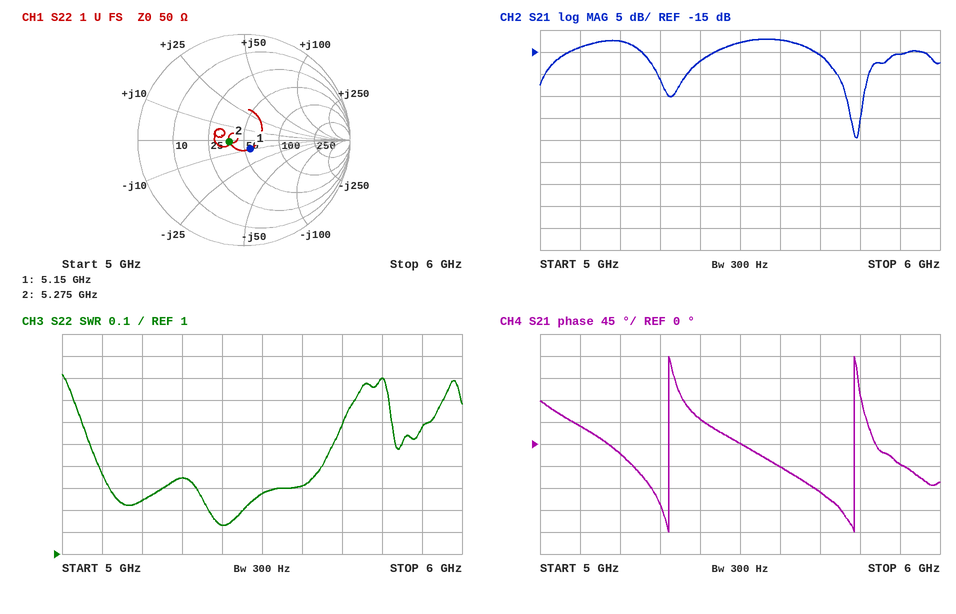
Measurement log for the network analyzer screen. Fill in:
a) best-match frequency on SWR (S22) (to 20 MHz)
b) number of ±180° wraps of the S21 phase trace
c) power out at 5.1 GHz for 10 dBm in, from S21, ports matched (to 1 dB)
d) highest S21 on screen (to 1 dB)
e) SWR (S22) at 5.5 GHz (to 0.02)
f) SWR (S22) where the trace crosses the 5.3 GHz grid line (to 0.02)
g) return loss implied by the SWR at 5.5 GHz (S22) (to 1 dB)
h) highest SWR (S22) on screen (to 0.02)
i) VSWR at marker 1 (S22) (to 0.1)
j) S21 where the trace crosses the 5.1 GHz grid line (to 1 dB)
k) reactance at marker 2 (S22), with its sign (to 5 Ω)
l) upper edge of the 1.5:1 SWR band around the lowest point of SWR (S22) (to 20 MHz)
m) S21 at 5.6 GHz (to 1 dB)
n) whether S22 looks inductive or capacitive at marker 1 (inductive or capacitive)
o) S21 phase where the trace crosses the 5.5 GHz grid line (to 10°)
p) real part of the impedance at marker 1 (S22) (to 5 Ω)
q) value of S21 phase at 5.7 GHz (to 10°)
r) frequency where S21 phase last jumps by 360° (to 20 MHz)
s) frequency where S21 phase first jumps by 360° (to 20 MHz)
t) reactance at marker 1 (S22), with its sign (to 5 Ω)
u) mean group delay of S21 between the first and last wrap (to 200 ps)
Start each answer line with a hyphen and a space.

- 5.40 GHz
- 2
- -4 dBm
- -12 dB
- 1.28
- 1.34
- 18 dB
- 1.82
- 1.2
- -14 dB
- 0 Ω
- 5.68 GHz
- -12 dB
- capacitive
- 0°
- 55 Ω
- -100°
- 5.78 GHz
- 5.32 GHz
- -10 Ω
- 2.2 ns
